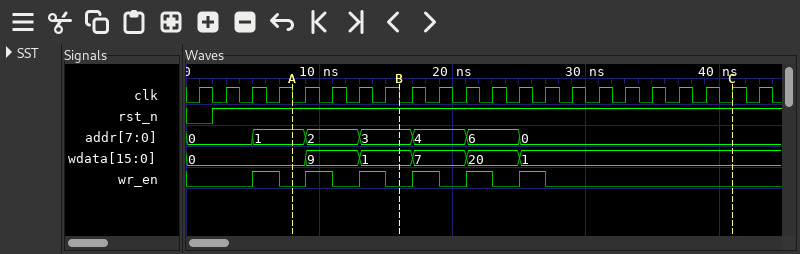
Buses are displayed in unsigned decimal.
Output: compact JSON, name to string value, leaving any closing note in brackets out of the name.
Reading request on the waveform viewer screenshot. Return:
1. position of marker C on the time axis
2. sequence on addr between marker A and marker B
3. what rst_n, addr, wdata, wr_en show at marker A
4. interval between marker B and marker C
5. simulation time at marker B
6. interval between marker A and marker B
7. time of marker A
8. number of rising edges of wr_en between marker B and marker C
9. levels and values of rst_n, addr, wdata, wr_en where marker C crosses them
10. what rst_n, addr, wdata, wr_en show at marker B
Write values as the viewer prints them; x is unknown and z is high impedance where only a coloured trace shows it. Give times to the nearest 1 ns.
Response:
{"position of marker C on the time axis": "41 ns", "sequence on addr between marker A and marker B": "1, 2, 3", "what rst_n, addr, wdata, wr_en show at marker A": "rst_n=1, addr=1, wdata=0, wr_en=0", "interval between marker B and marker C": "25 ns", "simulation time at marker B": "16 ns", "interval between marker A and marker B": "8 ns", "time of marker A": "8 ns", "number of rising edges of wr_en between marker B and marker C": "3", "levels and values of rst_n, addr, wdata, wr_en where marker C crosses them": "rst_n=1, addr=0, wdata=1, wr_en=0", "what rst_n, addr, wdata, wr_en show at marker B": "rst_n=1, addr=3, wdata=1, wr_en=0"}
